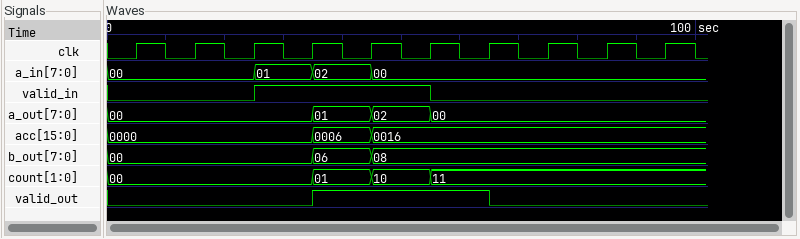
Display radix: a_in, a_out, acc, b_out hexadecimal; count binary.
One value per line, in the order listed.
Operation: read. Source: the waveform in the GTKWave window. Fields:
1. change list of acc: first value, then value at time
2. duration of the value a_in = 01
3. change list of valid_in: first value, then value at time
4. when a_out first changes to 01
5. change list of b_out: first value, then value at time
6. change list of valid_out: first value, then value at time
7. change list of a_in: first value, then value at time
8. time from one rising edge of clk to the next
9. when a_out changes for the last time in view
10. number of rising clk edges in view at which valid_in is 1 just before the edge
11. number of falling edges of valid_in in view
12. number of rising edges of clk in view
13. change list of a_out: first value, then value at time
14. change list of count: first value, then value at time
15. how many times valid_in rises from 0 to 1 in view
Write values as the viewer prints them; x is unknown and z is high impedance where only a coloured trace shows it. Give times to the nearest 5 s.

0000, 0006 at 35 s, 0016 at 45 s
10 s
0, 1 at 25 s, 0 at 55 s
35 s
00, 06 at 35 s, 08 at 45 s
0, 1 at 35 s, 0 at 65 s
00, 01 at 25 s, 02 at 35 s, 00 at 45 s
10 s
55 s
3
1
10
00, 01 at 35 s, 02 at 45 s, 00 at 55 s
00, 01 at 35 s, 10 at 45 s, 11 at 55 s
1
